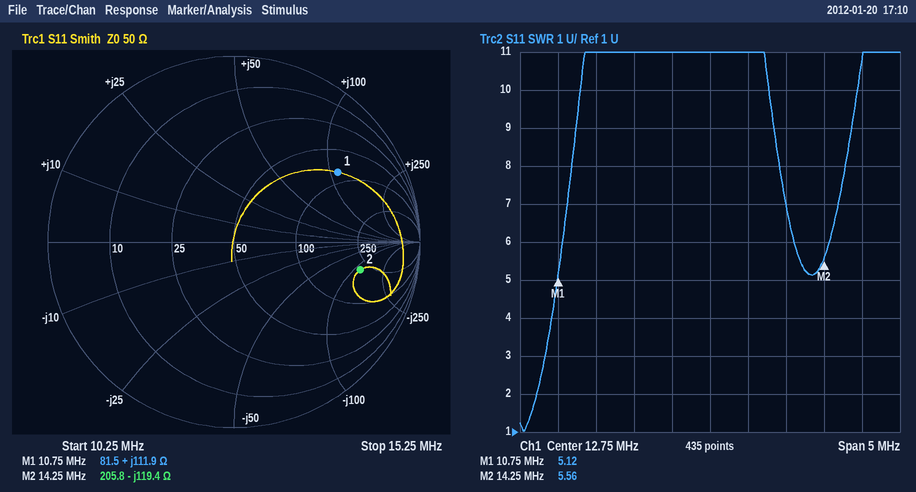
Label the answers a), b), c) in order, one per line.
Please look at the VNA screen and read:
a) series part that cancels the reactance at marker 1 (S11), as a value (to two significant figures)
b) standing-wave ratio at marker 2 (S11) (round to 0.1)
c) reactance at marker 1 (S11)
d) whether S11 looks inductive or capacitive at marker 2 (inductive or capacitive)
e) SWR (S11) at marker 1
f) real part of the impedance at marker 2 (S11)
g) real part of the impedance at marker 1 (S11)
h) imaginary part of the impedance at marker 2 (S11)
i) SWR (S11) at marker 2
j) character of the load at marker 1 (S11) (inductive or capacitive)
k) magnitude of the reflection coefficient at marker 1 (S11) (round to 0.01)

a) 130 pF
b) 5.6
c) +111.9 Ω
d) capacitive
e) 5.12
f) 205.8 Ω
g) 81.5 Ω
h) -119.4 Ω
i) 5.56
j) inductive
k) 0.67
